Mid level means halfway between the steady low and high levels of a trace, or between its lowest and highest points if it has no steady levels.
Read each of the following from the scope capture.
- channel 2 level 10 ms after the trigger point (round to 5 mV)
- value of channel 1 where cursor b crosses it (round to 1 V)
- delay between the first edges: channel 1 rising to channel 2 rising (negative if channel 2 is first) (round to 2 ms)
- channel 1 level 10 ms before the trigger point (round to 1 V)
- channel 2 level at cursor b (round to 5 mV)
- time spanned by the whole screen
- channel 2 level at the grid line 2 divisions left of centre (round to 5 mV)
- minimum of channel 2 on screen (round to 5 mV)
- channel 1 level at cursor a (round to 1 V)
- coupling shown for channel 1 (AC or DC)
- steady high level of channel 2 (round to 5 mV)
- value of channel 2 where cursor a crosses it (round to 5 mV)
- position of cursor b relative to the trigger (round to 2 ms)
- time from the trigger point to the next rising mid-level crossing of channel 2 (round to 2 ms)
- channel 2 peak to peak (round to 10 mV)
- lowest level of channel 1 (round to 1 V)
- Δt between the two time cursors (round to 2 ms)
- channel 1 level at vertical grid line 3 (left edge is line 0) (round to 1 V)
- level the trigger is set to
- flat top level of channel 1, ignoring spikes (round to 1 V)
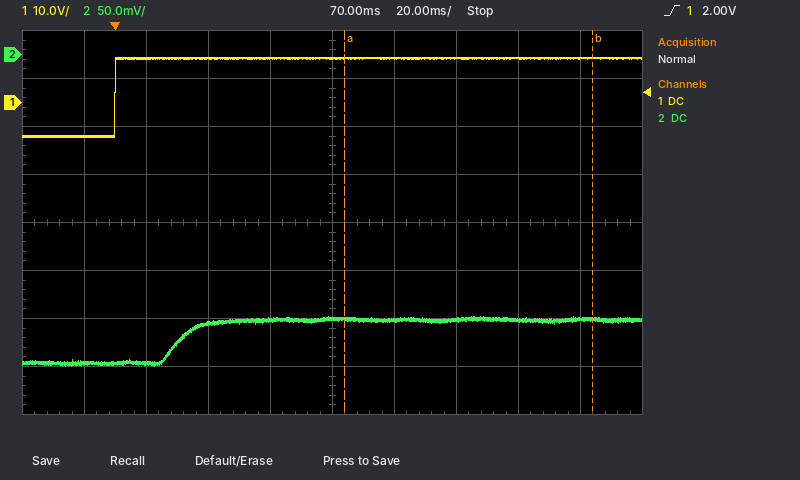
-320 mV
9 V
+20 ms
-7 V
-275 mV
200 ms
-280 mV
-325 mV
9 V
DC
-275 mV
-275 mV
+154 ms
20 ms
50 mV
-7 V
80 ms
9 V
2.00 V
9 V
